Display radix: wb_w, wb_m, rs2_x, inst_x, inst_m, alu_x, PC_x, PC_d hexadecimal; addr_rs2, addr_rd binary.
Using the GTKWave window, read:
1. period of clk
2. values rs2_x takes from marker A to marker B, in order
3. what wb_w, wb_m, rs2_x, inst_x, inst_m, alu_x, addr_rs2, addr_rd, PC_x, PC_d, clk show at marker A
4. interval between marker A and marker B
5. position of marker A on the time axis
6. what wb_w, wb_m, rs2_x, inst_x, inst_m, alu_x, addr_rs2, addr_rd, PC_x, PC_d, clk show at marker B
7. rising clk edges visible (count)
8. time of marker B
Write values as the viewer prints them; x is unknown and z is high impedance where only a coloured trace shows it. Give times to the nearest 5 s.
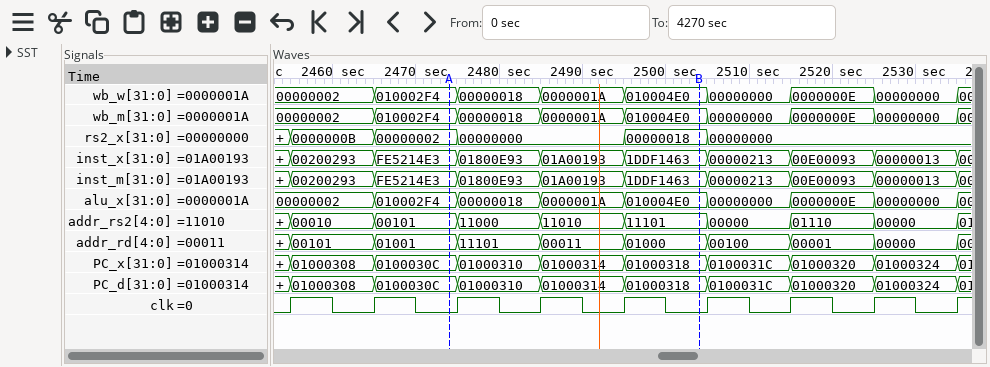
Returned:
10 s
00000002, 00000000, 00000018
wb_w=010002F4, wb_m=010002F4, rs2_x=00000002, inst_x=FE5214E3, inst_m=FE5214E3, alu_x=010002F4, addr_rs2=00101, addr_rd=01001, PC_x=0100030C, PC_d=0100030C, clk=0
30 s
2475 s
wb_w=010004E0, wb_m=010004E0, rs2_x=00000018, inst_x=1DDF1463, inst_m=1DDF1463, alu_x=010004E0, addr_rs2=11101, addr_rd=01000, PC_x=01000318, PC_d=01000318, clk=0
9
2505 s
